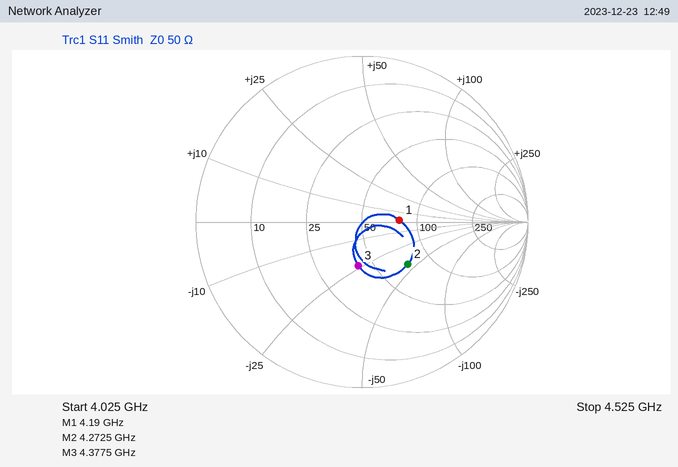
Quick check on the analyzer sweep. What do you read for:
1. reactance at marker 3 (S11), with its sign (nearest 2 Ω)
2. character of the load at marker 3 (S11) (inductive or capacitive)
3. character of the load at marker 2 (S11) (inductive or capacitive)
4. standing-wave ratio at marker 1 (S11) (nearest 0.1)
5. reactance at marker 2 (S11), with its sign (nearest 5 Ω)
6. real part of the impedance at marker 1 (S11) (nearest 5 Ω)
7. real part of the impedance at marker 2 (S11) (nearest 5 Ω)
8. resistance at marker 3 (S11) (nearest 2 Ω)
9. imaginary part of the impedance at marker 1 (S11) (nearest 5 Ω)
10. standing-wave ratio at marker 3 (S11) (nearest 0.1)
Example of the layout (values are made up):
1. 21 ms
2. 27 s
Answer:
1. -24 Ω
2. capacitive
3. capacitive
4. 1.6
5. -45 Ω
6. 80 Ω
7. 75 Ω
8. 42 Ω
9. 0 Ω
10. 1.7
